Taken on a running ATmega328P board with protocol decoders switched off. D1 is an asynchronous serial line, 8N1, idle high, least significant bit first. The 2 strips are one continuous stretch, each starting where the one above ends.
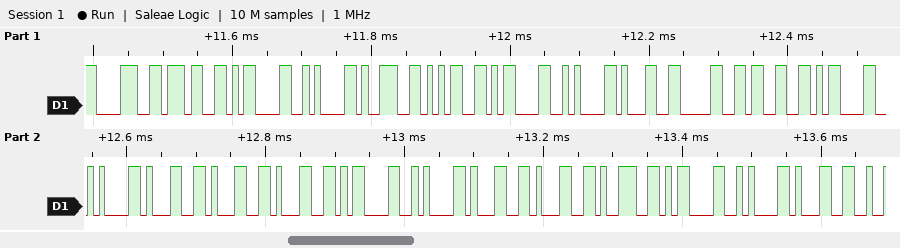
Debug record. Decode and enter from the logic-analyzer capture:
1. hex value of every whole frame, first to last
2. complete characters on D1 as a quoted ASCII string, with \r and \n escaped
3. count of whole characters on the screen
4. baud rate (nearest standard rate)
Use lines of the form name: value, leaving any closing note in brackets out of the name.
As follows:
hex value of every whole frame, first to last: 38 37 0D 0A 39 35 0D 0A 31 30 33 0D 0A 31 31 31 0D 0A 31 31 39 0D 0A 31
complete characters on D1 as a quoted ASCII string, with \r and \n escaped: "87\r\n95\r\n103\r\n111\r\n119\r\n1"
count of whole characters on the screen: 24
baud rate: 115200 baud
